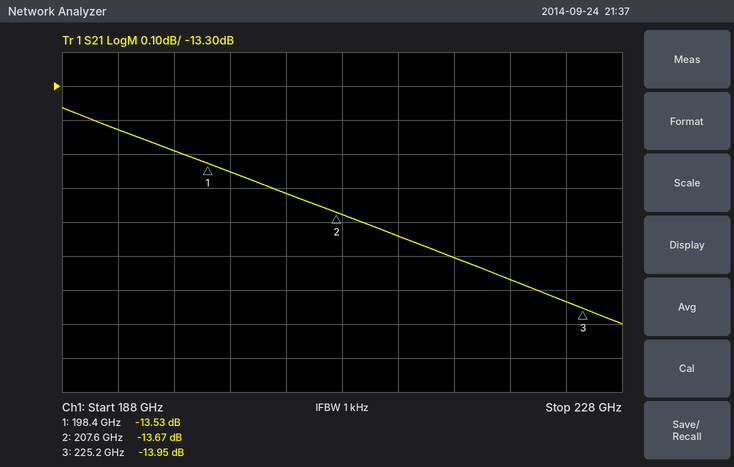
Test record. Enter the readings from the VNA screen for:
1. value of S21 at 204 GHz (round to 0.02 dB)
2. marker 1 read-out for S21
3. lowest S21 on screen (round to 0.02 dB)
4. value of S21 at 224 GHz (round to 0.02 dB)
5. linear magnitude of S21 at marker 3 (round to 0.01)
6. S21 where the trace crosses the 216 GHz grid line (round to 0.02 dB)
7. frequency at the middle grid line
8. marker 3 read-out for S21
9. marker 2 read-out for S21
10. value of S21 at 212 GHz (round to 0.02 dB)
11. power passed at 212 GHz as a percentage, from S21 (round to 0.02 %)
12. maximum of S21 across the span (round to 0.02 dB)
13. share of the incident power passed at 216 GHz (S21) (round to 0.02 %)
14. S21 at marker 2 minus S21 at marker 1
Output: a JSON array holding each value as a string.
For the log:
["-13.62 dB", "-13.53 dB", "-14.00 dB", "-13.94 dB", "0.20", "-13.80 dB", "208 GHz", "-13.95 dB", "-13.67 dB", "-13.74 dB", "4.22 %", "-13.36 dB", "4.16 %", "-0.14 dB"]
